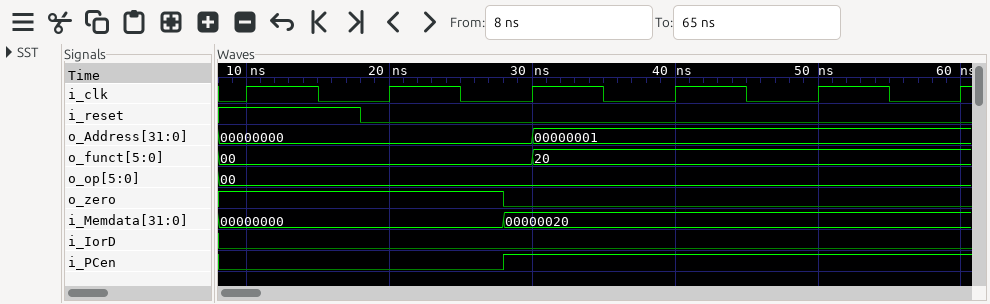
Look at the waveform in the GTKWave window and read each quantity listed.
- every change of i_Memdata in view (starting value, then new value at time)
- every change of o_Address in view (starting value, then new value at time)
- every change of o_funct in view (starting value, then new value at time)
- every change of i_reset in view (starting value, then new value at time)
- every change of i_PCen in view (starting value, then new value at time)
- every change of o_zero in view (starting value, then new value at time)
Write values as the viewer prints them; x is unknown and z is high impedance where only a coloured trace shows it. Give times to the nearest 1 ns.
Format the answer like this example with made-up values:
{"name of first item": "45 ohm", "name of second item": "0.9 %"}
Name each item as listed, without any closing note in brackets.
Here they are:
{"every change of i_Memdata in view": "00000000, 00000020 at 28 ns", "every change of o_Address in view": "00000000, 00000001 at 30 ns", "every change of o_funct in view": "00, 20 at 30 ns", "every change of i_reset in view": "1, 0 at 18 ns", "every change of i_PCen in view": "0, 1 at 28 ns", "every change of o_zero in view": "1, 0 at 28 ns"}
